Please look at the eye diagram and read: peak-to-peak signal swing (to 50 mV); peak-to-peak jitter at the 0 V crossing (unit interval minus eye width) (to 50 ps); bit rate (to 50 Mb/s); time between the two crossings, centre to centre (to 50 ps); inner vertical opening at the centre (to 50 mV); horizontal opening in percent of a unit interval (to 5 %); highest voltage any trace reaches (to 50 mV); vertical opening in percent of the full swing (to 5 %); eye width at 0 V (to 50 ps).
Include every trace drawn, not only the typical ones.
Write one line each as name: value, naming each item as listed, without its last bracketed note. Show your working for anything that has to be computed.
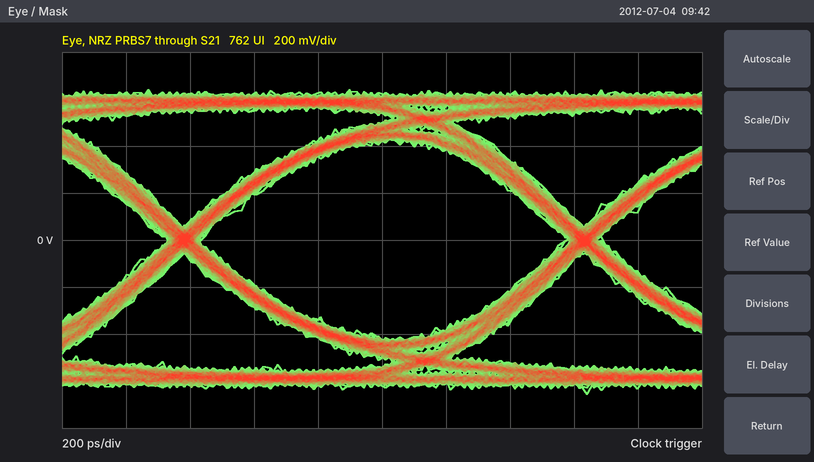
peak-to-peak signal swing: 1.30 V
peak-to-peak jitter at the 0 V crossing (unit interval minus eye width): 100 ps
bit rate: 800 Mb/s
time between the two crossings, centre to centre: 1.25 ns
inner vertical opening at the centre: 850 mV
horizontal opening in percent of a unit interval: 1.15 ns / 1.25 ns ≈ 92.0 %, so 90 % to the nearest 5 %
highest voltage any trace reaches: 650 mV
vertical opening in percent of the full swing: 850 mV / 1.30 V ≈ 65 %
eye width at 0 V: 1.15 ns
